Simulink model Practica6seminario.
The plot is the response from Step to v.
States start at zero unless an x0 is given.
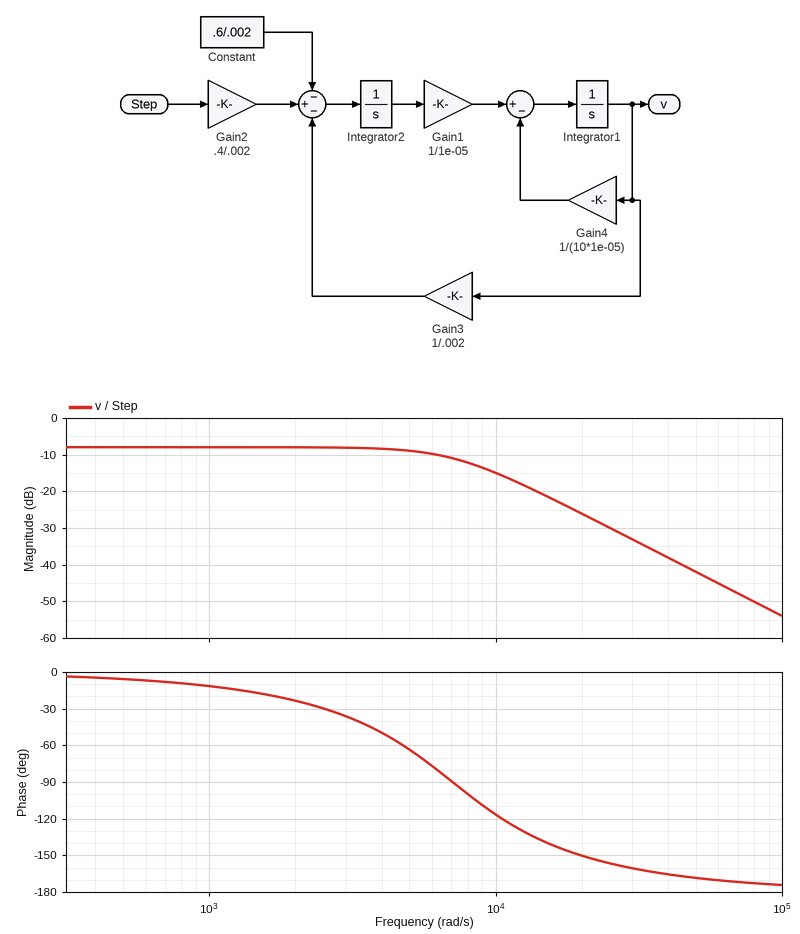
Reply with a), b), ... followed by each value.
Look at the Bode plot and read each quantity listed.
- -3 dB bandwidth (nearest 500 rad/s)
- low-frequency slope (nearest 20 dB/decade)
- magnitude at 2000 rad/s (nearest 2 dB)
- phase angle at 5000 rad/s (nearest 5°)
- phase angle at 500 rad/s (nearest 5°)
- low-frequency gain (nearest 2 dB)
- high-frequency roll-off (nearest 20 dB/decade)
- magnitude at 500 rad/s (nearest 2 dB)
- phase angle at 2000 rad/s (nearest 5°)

a) 7000 rad/s
b) 0 dB/decade
c) -8 dB
d) -65°
e) -5°
f) -8 dB
g) -40 dB/decade
h) -8 dB
i) -25°
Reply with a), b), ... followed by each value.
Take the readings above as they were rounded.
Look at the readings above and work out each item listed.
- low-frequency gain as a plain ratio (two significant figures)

a) 0.40
